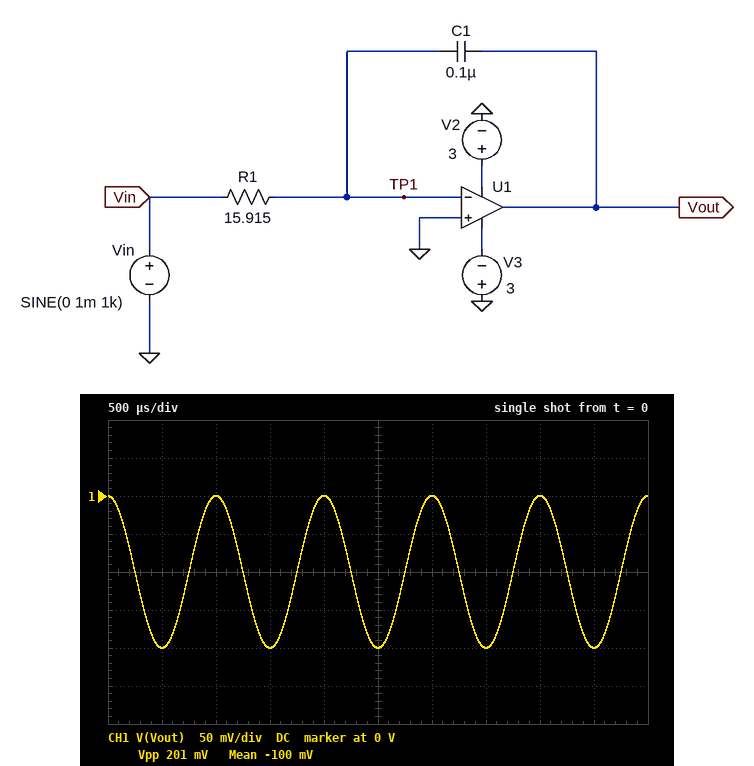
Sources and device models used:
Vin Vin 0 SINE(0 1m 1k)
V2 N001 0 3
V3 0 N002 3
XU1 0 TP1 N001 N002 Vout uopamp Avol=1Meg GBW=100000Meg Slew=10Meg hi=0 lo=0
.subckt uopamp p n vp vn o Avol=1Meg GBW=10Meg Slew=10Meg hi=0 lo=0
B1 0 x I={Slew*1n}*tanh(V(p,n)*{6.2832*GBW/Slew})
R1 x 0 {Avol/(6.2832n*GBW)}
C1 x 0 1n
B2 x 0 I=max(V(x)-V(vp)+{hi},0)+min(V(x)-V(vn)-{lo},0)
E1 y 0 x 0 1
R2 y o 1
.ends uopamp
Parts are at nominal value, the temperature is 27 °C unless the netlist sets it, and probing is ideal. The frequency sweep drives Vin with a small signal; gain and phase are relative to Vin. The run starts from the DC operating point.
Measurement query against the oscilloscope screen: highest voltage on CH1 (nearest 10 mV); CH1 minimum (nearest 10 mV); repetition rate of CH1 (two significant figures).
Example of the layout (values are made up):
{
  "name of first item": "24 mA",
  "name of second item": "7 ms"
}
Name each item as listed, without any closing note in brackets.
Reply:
{
  "highest voltage on CH1": "0 V",
  "CH1 minimum": "-200 mV",
  "repetition rate of CH1": "1.0 kHz"
}
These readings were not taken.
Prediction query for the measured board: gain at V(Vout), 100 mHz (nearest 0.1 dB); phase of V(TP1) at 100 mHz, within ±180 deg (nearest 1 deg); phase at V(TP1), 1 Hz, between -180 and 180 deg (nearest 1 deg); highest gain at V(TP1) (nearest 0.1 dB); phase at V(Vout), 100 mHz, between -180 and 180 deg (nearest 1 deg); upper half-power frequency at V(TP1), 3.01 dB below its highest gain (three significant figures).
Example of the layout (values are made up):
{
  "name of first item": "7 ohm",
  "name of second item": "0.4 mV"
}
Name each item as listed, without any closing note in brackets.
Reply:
{
  "gain at V(Vout), 100 mHz": "117.0 dB",
  "phase of V(TP1) at 100 mHz, within ±180 deg": "-45 deg",
  "phase at V(TP1), 1 Hz, between -180 and 180 deg": "-84 deg",
  "highest gain at V(TP1)": "0 dB",
  "phase at V(Vout), 100 mHz, between -180 and 180 deg": "135 deg",
  "upper half-power frequency at V(TP1), 3.01 dB below its highest gain": "100 mHz"
}
